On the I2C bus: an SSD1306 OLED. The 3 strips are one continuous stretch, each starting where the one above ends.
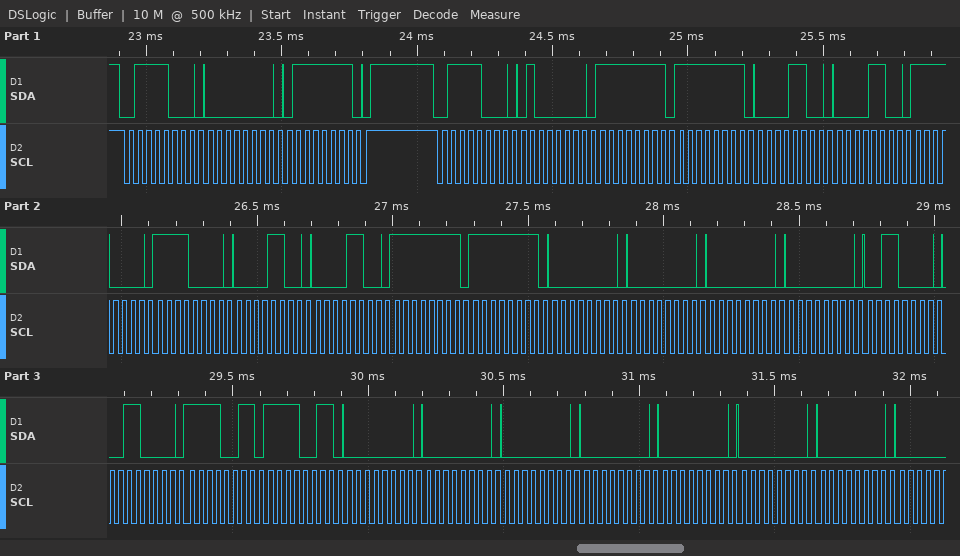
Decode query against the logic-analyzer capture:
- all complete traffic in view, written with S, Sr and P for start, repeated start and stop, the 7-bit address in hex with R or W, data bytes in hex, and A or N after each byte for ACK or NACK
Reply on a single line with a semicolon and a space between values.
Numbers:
S 3CW A 00 A 7F A P S 3CW A 40 A FF A FF A 0C A 0C A F0 A F0 A 0C A 0C A FF A FF A 00 A 00 A 00 A 00 A 30 A 30 A F3 A F3 A 00 A 00 A 00 A 00 A 00 A 00 A 00 A
